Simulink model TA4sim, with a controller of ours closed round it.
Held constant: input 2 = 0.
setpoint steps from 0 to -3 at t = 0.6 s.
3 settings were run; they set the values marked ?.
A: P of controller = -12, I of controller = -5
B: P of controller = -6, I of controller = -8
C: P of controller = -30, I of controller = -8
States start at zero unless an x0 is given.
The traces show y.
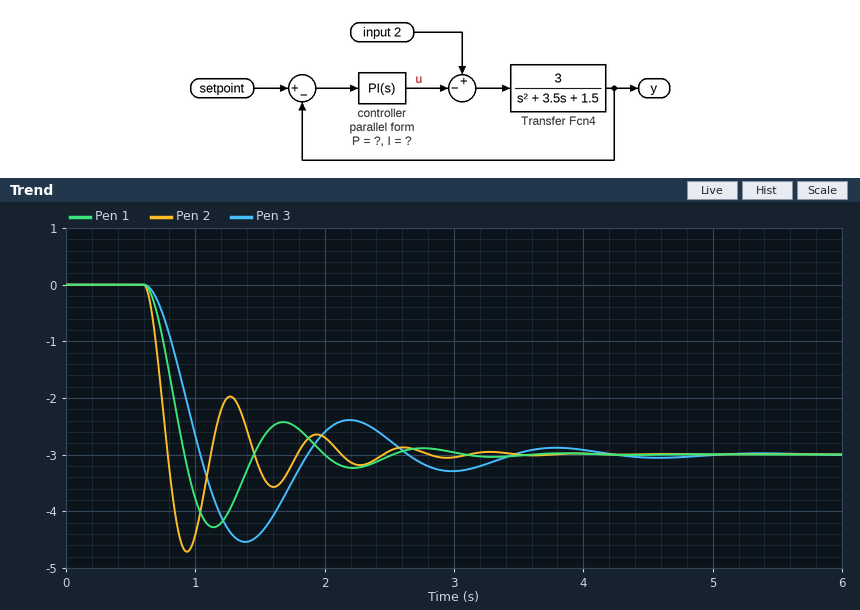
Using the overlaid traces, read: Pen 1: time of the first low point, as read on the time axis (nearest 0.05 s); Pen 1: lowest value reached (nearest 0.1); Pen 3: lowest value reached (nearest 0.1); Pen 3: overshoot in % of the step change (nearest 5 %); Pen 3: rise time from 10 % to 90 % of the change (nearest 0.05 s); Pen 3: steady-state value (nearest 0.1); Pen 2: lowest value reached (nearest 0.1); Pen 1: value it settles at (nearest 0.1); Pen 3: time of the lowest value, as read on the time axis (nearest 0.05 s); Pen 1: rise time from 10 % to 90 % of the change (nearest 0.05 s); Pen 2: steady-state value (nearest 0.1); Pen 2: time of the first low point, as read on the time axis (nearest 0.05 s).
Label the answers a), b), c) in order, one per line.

a) 1.15 s
b) -4.3
c) -4.5
d) 50 %
e) 0.30 s
f) -3.0
g) -4.7
h) -3.0
i) 1.40 s
j) 0.20 s
k) -3.0
l) 0.95 s
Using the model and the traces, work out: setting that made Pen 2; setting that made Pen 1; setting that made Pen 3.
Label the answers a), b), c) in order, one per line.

a) C
b) A
c) B
